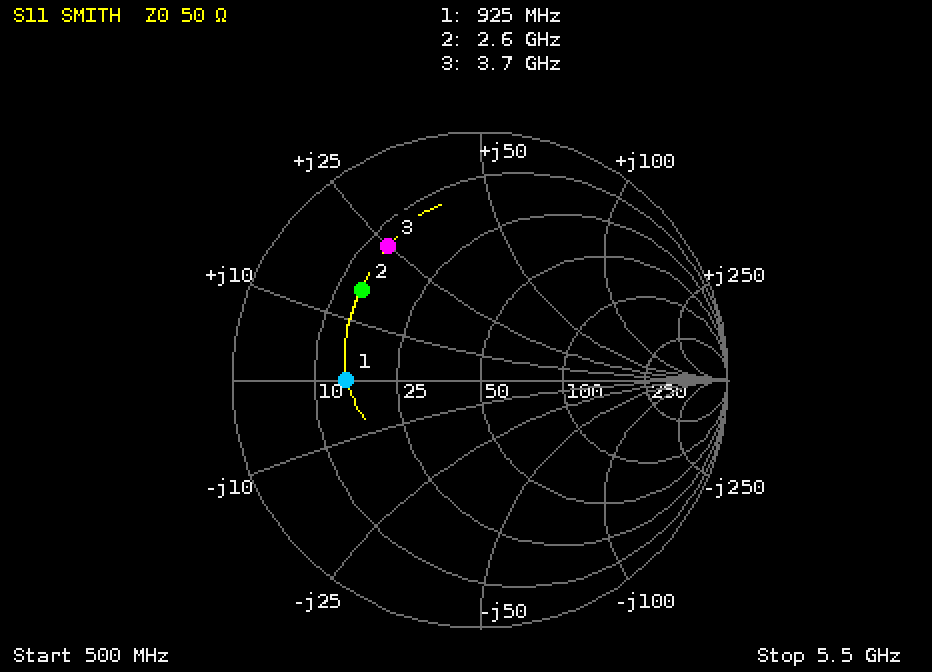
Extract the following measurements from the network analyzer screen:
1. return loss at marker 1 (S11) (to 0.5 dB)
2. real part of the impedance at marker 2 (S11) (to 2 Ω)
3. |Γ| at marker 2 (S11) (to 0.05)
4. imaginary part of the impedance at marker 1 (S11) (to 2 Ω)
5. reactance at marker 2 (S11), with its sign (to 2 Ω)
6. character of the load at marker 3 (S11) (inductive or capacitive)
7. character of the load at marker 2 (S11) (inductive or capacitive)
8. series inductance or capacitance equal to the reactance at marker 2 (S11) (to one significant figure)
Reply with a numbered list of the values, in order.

1. 5.5 dB
2. 14 Ω
3. 0.60
4. 0 Ω
5. +16 Ω
6. inductive
7. inductive
8. 1.0 nH
